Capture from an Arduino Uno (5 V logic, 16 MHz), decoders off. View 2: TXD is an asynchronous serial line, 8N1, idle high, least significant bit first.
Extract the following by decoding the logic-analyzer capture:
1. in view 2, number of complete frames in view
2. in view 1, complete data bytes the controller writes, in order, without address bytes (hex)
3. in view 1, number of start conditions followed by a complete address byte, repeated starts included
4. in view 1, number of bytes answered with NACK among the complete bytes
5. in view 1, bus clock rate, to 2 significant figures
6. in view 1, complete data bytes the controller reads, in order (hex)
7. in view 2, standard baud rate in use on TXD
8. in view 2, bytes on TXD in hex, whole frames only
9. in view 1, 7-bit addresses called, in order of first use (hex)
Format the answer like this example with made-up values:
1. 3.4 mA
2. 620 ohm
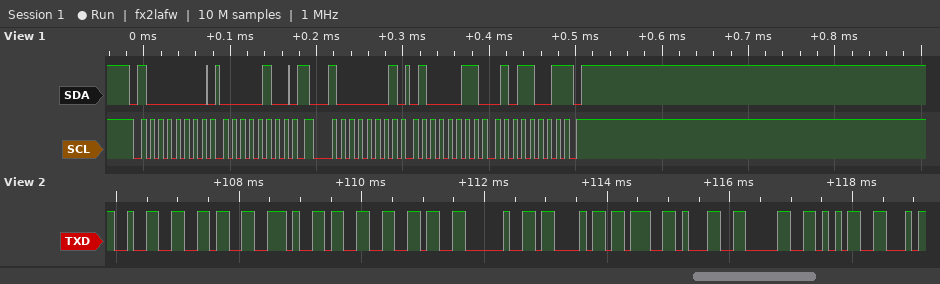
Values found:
1. 11
2. 04
3. 2
4. 1
5. 100 kHz
6. 43 59
7. 9600 baud
8. 32 36 2E 33 36 20 43 3B 31 30 35
9. 0x40
